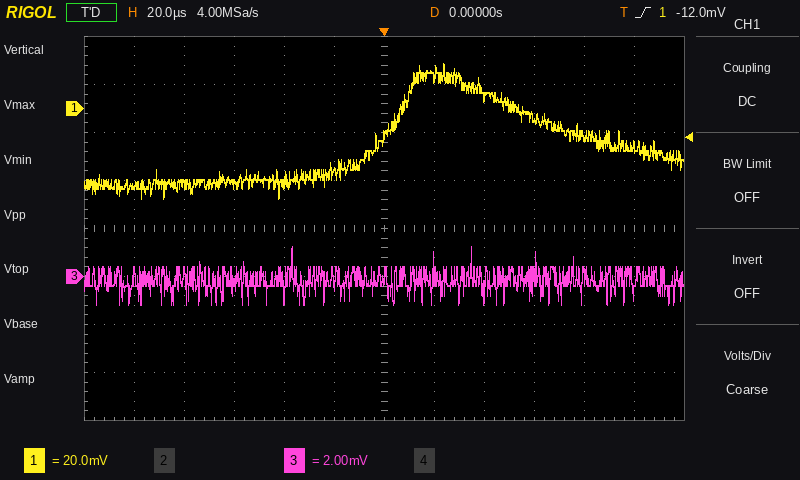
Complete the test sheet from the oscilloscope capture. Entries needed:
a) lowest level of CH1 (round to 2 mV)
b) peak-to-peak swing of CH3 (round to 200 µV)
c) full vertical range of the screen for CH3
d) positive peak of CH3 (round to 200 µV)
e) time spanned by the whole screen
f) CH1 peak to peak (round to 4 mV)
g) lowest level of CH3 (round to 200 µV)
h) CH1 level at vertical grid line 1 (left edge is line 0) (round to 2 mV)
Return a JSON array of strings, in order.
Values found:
["-38 mV", "2.4 mV", "16 mV", "1.2 mV", "240 µs", "56 mV", "-1.2 mV", "-32 mV"]
